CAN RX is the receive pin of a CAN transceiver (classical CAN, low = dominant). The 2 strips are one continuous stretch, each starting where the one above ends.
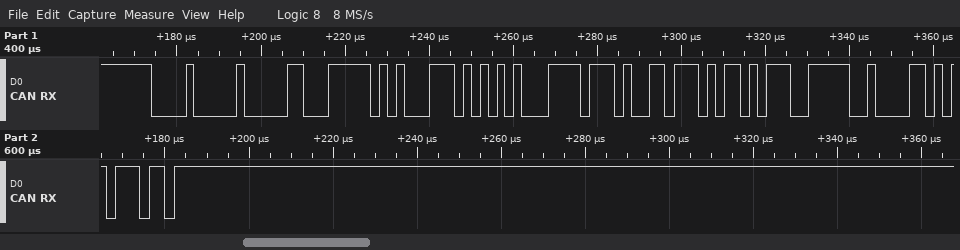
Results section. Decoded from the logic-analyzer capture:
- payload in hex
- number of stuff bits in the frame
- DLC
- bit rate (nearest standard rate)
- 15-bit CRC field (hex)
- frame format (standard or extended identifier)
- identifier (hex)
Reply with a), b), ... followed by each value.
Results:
a) FD 1D 54 7B A6 EB 5C FA
b) 4
c) 8
d) 500 kbit/s
e) 0x0D5D
f) standard
g) 0x080
